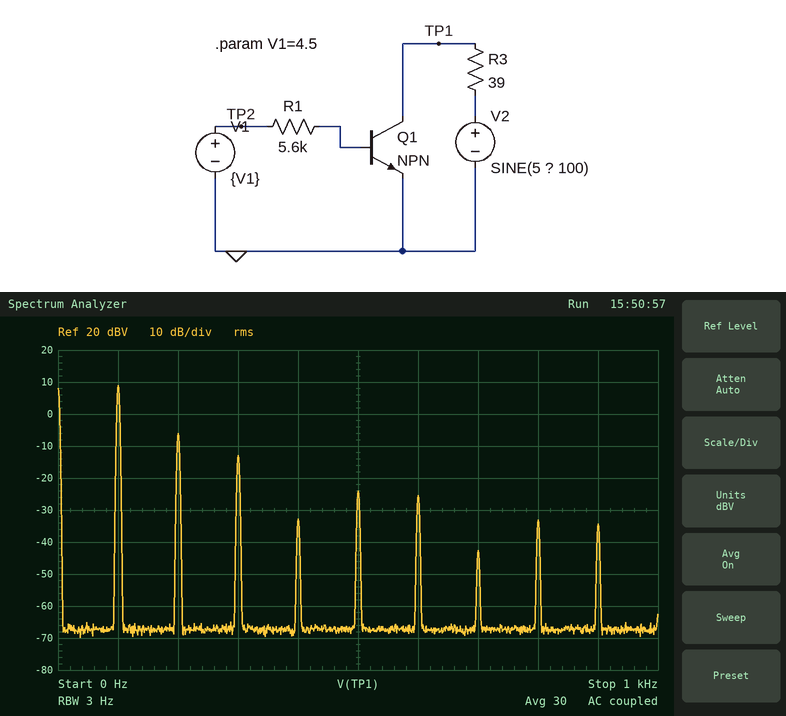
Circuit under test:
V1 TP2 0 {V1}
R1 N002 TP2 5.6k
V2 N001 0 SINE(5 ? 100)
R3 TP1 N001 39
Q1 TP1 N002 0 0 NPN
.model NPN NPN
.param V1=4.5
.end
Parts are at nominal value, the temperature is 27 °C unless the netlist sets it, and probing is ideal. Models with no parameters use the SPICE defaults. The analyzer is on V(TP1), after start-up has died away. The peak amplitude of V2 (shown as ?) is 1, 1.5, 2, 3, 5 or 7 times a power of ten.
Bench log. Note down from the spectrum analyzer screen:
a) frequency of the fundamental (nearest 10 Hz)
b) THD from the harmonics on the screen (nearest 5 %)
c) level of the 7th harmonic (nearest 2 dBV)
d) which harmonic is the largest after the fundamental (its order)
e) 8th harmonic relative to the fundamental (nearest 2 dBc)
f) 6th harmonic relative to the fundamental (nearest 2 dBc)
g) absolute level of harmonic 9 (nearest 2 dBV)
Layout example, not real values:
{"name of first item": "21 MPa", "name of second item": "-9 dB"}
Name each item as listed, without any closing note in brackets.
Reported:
{"frequency of the fundamental": "100 Hz", "THD from the harmonics on the screen": "20 %", "level of the 7th harmonic": "-42 dBV", "which harmonic is the largest after the fundamental": "2", "8th harmonic relative to the fundamental": "-42 dBc", "6th harmonic relative to the fundamental": "-34 dBc", "absolute level of harmonic 9": "-34 dBV"}
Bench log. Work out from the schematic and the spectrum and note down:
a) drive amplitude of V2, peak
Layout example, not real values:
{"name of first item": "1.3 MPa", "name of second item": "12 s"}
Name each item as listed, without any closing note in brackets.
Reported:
{"drive amplitude of V2, peak": "5 V"}
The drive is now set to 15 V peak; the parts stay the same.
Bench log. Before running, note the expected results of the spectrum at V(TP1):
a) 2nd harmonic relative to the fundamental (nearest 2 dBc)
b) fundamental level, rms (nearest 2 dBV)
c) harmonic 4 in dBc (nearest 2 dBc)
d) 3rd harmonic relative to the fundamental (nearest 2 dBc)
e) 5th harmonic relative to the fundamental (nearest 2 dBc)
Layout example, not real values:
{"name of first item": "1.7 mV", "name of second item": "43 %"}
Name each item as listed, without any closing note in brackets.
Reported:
{"2nd harmonic relative to the fundamental": "-30 dBc", "fundamental level, rms": "20 dBV", "harmonic 4 in dBc": "-32 dBc", "3rd harmonic relative to the fundamental": "-30 dBc", "5th harmonic relative to the fundamental": "-42 dBc"}
